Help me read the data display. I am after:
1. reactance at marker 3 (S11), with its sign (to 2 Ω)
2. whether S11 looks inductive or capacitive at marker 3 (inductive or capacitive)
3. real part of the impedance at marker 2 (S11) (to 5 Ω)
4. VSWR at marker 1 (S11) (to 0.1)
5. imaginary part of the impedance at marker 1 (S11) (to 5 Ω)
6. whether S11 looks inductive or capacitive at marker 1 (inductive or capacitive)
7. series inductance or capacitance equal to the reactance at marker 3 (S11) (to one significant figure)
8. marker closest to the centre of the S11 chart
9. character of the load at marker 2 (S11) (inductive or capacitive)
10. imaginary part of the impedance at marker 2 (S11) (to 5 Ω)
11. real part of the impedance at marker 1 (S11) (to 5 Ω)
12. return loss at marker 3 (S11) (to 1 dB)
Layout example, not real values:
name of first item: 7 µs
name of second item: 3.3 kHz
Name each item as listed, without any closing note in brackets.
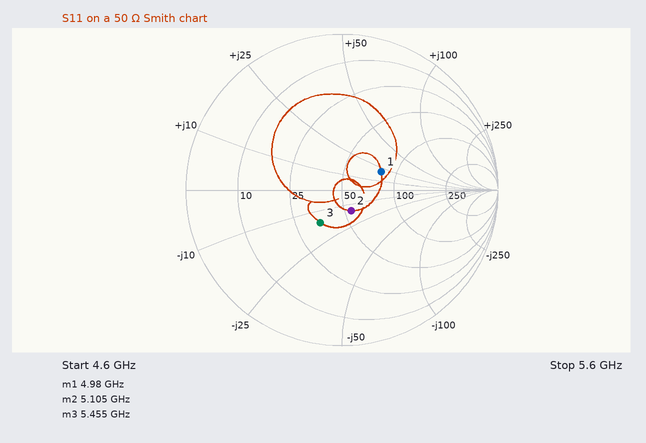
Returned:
reactance at marker 3 (S11), with its sign: -16 Ω
whether S11 looks inductive or capacitive at marker 3: capacitive
real part of the impedance at marker 2 (S11): 55 Ω
VSWR at marker 1 (S11): 1.8
imaginary part of the impedance at marker 1 (S11): +20 Ω
whether S11 looks inductive or capacitive at marker 1: inductive
series inductance or capacitance equal to the reactance at marker 3 (S11): 2 pF
marker closest to the centre of the S11 chart: marker 2
character of the load at marker 2 (S11): capacitive
imaginary part of the impedance at marker 2 (S11): -15 Ω
real part of the impedance at marker 1 (S11): 80 Ω
return loss at marker 3 (S11): 12 dB
